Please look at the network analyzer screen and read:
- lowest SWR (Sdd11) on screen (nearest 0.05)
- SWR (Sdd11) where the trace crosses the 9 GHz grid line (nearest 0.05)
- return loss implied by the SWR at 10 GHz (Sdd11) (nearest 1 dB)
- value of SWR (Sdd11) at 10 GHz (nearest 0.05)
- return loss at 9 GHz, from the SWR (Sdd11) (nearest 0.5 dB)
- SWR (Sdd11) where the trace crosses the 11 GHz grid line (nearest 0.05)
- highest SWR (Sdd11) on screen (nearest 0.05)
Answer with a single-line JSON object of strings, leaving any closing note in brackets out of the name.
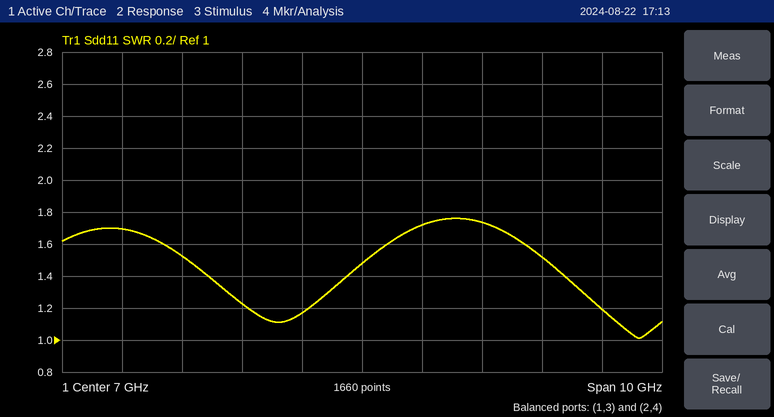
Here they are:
{"lowest SWR (Sdd11) on screen": "1.00", "SWR (Sdd11) where the trace crosses the 9 GHz grid line": "1.75", "return loss implied by the SWR at 10 GHz (Sdd11)": "14 dB", "value of SWR (Sdd11) at 10 GHz": "1.50", "return loss at 9 GHz, from the SWR (Sdd11)": "11.5 dB", "SWR (Sdd11) where the trace crosses the 11 GHz grid line": "1.20", "highest SWR (Sdd11) on screen": "1.75"}
